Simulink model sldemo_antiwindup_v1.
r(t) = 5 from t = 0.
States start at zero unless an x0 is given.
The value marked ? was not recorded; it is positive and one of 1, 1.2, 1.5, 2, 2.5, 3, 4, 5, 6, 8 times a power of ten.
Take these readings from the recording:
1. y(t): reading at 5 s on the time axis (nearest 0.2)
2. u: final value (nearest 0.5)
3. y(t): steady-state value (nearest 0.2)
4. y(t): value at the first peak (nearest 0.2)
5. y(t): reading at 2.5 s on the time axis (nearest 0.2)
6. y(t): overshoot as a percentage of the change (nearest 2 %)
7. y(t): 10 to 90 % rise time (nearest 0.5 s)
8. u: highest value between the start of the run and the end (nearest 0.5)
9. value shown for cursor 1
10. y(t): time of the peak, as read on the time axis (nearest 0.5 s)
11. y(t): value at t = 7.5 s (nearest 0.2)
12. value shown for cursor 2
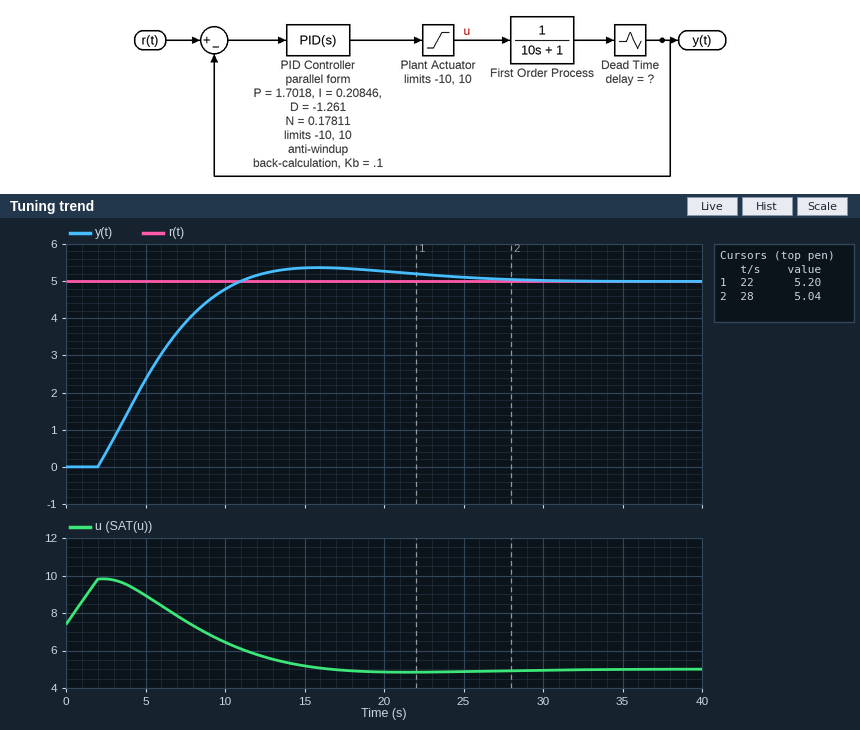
2.4
5.0
5.0
5.4
0.4
8 %
6.5 s
10.0
5.20
16.0 s
3.8
5.04
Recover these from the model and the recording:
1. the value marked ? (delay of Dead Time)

2
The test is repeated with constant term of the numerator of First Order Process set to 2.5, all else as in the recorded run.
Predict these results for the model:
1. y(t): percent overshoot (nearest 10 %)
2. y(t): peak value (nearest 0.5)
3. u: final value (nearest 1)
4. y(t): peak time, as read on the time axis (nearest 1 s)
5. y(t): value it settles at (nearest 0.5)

40 %
7.0
2
7 s
5.0
